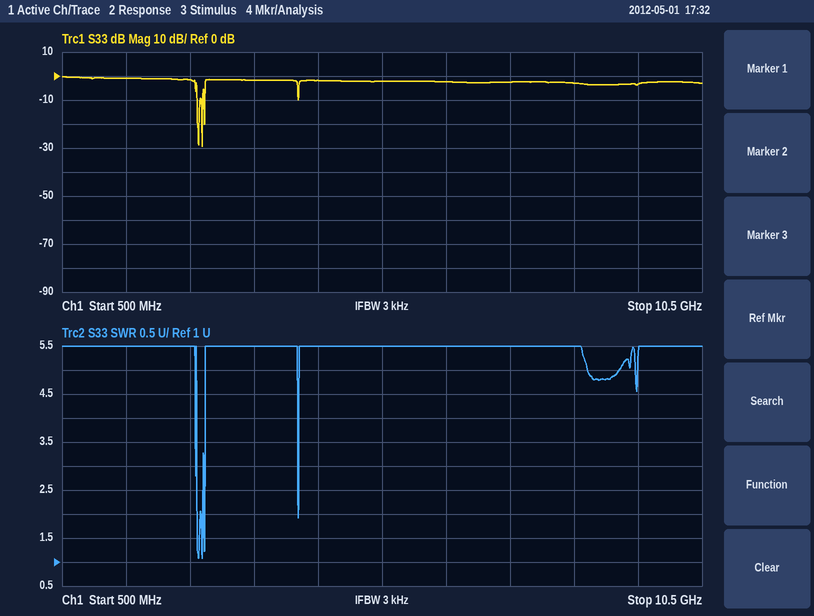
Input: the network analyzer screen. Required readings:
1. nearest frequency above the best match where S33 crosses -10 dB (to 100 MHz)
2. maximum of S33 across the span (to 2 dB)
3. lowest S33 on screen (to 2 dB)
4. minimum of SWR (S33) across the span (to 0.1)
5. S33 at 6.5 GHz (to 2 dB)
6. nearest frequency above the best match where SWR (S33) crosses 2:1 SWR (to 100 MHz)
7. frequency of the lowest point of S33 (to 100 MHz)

2.7 GHz
0 dB
-30 dB
1.1
-2 dB
2.7 GHz
2.7 GHz
